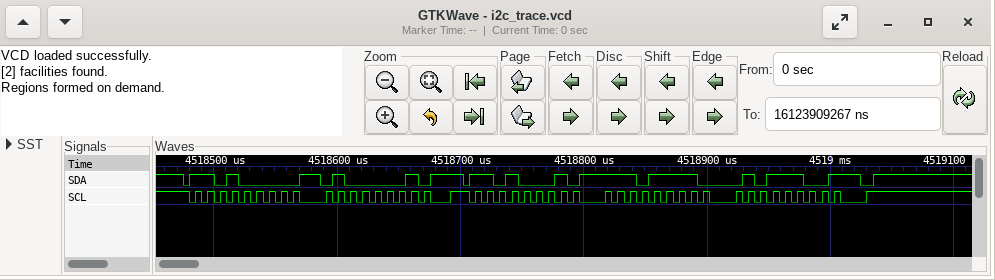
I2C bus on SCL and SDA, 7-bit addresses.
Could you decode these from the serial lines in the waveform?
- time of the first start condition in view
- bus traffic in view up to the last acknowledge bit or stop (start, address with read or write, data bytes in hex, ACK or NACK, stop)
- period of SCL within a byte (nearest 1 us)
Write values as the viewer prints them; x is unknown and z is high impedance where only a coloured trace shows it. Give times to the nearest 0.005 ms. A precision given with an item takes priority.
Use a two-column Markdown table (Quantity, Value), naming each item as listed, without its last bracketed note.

| Quantity | Value |
|---|---|
| time of the first start condition in view | 4518.475 ms |
| bus traffic in view up to the last acknowledge bit or stop | start, address 68 write ACK, 41 ACK, repeated start, address 68 read ACK, EF ACK, 5C NACK, stop |
| period of SCL within a byte | 10 us |
